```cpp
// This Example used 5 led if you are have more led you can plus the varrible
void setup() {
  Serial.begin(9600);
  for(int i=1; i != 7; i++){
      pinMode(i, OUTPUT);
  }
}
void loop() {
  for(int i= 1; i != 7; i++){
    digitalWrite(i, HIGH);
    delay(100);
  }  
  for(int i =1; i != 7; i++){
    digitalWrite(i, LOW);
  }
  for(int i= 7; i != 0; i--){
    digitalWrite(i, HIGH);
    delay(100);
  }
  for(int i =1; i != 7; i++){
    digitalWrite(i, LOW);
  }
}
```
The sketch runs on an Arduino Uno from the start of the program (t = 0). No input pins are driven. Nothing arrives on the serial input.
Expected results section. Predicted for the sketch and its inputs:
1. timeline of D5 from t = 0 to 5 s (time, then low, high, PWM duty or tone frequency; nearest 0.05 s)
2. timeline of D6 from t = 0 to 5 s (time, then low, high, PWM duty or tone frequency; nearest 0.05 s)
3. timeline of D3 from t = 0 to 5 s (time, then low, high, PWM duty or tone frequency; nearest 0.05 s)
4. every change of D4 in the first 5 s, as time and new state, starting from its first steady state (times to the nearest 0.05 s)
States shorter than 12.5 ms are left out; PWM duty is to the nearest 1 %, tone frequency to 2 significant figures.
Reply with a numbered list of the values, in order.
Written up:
1. 0 s low; 0.4 s high; 0.6 s low; 0.8 s high; 1.3 s low; 1.7 s high; 1.9 s low; 2.1 s high; 2.6 s low; 3 s high; 3.2 s low; 3.4 s high; 3.9 s low; 4.3 s high; 4.5 s low; 4.7 s high
2. 0 s low; 0.5 s high; 0.6 s low; 0.7 s high; 1.3 s low; 1.8 s high; 1.9 s low; 2 s high; 2.6 s low; 3.1 s high; 3.2 s low; 3.3 s high; 3.9 s low; 4.4 s high; 4.5 s low; 4.6 s high
3. 0 s low; 0.2 s high; 0.6 s low; 1 s high; 1.3 s low; 1.5 s high; 1.9 s low; 2.3 s high; 2.6 s low; 2.8 s high; 3.2 s low; 3.6 s high; 3.9 s low; 4.1 s high; 4.5 s low; 4.9 s high
4. 0 s low; 0.3 s high; 0.6 s low; 0.9 s high; 1.3 s low; 1.6 s high; 1.9 s low; 2.2 s high; 2.6 s low; 2.9 s high; 3.2 s low; 3.5 s high; 3.9 s low; 4.2 s high; 4.5 s low; 4.8 s high
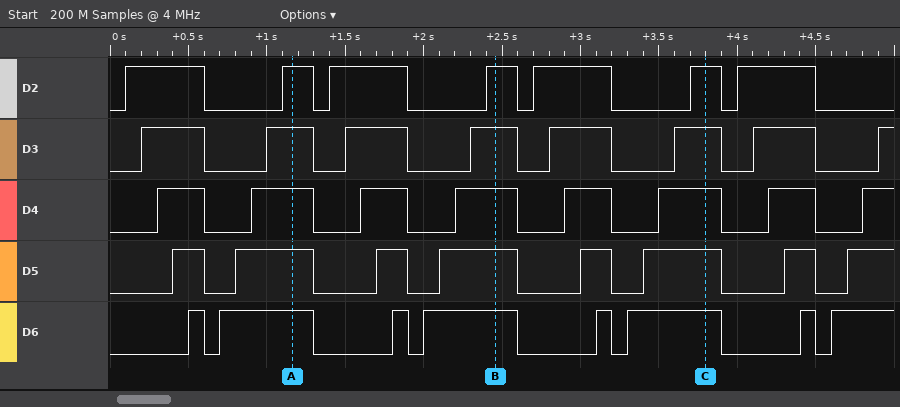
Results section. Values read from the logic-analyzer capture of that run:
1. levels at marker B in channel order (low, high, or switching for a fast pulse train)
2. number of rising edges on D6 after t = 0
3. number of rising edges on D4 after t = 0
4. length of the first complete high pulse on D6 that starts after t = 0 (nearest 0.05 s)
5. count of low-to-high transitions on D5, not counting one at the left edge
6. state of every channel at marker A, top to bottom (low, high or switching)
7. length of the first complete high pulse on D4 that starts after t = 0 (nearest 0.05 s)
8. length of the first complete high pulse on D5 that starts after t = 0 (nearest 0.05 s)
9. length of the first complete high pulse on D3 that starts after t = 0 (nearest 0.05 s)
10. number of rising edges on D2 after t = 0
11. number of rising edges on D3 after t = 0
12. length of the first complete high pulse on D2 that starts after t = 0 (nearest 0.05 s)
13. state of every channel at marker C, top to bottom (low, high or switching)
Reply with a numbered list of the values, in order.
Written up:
1. D2 high, D3 high, D4 high, D5 high, D6 high
2. 8
3. 8
4. 0.10 s
5. 8
6. D2 high, D3 high, D4 high, D5 high, D6 high
7. 0.30 s
8. 0.20 s
9. 0.40 s
10. 7
11. 8
12. 0.50 s
13. D2 high, D3 high, D4 high, D5 high, D6 high
